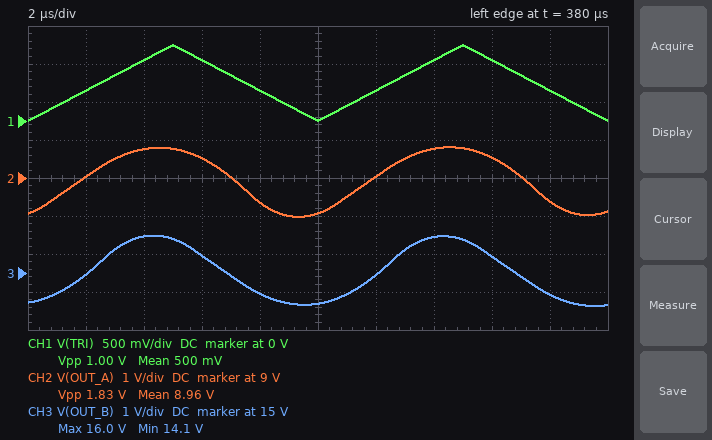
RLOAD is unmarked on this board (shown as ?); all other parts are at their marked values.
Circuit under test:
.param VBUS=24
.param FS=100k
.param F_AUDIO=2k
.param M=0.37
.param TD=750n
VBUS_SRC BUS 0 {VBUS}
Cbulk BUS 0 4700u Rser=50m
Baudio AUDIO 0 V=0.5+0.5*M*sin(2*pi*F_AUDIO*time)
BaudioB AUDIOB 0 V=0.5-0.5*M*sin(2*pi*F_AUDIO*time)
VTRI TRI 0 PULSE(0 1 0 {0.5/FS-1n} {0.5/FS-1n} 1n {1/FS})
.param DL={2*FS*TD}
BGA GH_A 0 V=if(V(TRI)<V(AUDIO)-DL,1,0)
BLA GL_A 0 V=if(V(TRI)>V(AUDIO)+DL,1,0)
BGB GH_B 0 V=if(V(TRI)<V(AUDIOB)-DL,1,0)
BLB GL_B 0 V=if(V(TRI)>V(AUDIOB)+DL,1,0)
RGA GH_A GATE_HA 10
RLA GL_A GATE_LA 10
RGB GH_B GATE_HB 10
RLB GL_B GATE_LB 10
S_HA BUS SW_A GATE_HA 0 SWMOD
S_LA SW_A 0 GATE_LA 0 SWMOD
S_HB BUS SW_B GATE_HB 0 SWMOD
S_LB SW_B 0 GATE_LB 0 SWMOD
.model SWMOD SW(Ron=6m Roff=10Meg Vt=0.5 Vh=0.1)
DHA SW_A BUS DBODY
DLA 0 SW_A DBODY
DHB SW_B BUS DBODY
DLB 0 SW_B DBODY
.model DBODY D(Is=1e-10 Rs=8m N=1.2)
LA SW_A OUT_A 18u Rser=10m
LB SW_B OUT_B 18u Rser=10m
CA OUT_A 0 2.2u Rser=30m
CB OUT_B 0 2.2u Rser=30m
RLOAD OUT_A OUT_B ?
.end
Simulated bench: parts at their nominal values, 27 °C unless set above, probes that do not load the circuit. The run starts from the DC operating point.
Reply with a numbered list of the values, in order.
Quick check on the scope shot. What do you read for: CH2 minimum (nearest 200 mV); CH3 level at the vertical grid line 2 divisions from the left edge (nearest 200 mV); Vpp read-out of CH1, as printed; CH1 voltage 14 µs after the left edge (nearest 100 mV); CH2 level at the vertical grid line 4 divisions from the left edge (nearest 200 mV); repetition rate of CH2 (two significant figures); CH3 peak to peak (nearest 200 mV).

1. 8.0 V
2. 16.0 V
3. 1.00 V
4. 800 mV
5. 8.4 V
6. 100 kHz
7. 1.8 V
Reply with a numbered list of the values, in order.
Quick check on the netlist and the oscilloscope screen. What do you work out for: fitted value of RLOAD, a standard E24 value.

1. 5.1 Ω
